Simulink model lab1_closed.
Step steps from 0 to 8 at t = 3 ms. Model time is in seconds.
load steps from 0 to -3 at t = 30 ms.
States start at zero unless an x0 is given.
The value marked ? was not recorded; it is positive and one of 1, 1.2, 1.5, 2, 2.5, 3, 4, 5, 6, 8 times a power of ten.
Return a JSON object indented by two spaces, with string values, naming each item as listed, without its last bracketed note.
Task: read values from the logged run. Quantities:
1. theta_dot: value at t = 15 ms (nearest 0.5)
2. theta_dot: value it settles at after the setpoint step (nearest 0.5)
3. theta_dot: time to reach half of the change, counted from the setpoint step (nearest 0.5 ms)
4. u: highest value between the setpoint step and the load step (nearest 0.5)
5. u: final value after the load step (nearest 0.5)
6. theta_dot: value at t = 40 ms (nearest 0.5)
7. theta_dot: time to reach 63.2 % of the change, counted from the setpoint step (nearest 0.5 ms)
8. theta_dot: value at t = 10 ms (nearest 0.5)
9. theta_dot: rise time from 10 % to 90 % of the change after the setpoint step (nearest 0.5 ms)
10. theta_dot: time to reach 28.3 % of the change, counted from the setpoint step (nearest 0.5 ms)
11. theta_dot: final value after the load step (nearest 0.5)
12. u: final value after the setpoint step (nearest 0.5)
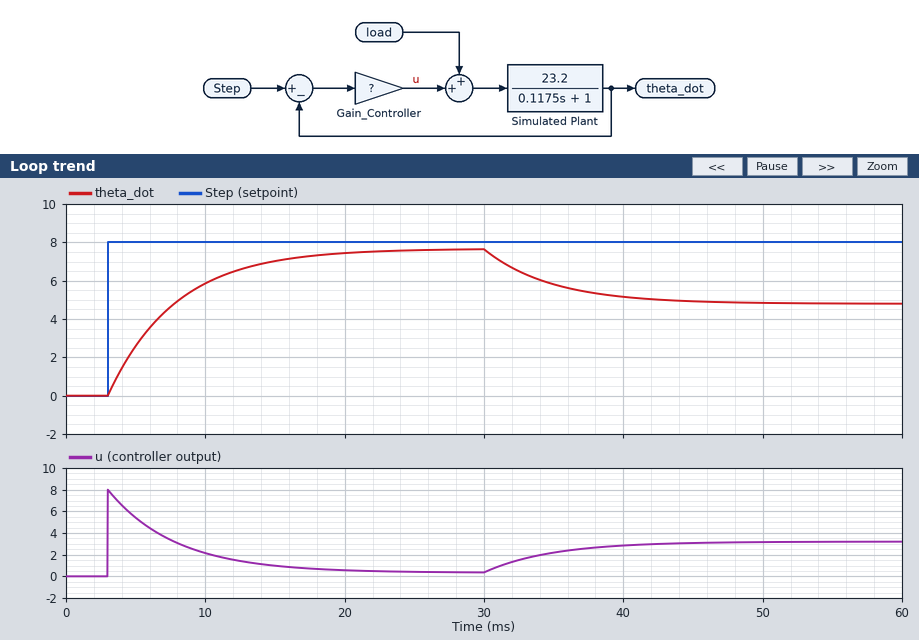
{
  "theta_dot: value at t = 15 ms": "7.0",
  "theta_dot: value it settles at after the setpoint step": "7.5",
  "theta_dot: time to reach half of the change, counted from the setpoint step": "3.5 ms",
  "u: highest value between the setpoint step and the load step": "8.0",
  "u: final value after the load step": "3.0",
  "theta_dot: value at t = 40 ms": "5.0",
  "theta_dot: time to reach 63.2 % of the change, counted from the setpoint step": "5.0 ms",
  "theta_dot: value at t = 10 ms": "6.0",
  "theta_dot: rise time from 10 % to 90 % of the change after the setpoint step": "10.5 ms",
  "theta_dot: time to reach 28.3 % of the change, counted from the setpoint step": "1.5 ms",
  "theta_dot: final value after the load step": "5.0",
  "u: final value after the setpoint step": "0.5"
}
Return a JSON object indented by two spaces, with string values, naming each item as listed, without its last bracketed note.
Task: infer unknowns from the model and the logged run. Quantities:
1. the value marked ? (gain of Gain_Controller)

{
  "the value marked ?": "1"
}
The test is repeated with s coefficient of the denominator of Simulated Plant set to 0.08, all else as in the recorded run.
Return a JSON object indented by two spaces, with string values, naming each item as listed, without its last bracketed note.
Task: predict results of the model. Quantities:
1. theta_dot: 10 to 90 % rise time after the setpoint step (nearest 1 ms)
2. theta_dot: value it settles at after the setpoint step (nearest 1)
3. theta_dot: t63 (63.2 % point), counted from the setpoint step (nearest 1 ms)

{
  "theta_dot: 10 to 90 % rise time after the setpoint step": "7 ms",
  "theta_dot: value it settles at after the setpoint step": "8",
  "theta_dot: t63 (63.2 % point), counted from the setpoint step": "3 ms"
}
